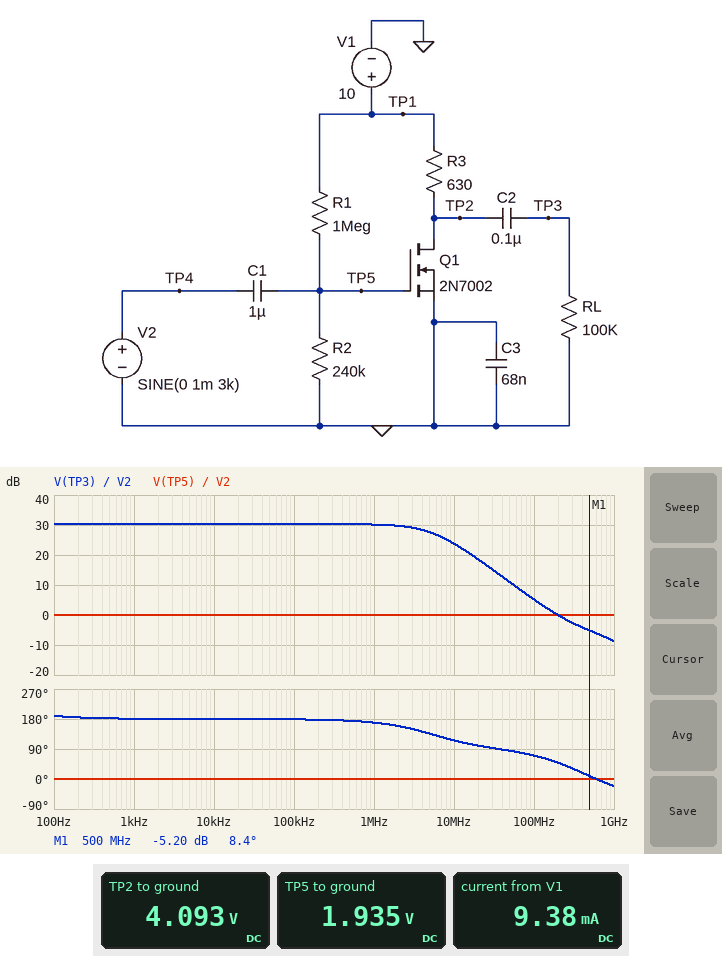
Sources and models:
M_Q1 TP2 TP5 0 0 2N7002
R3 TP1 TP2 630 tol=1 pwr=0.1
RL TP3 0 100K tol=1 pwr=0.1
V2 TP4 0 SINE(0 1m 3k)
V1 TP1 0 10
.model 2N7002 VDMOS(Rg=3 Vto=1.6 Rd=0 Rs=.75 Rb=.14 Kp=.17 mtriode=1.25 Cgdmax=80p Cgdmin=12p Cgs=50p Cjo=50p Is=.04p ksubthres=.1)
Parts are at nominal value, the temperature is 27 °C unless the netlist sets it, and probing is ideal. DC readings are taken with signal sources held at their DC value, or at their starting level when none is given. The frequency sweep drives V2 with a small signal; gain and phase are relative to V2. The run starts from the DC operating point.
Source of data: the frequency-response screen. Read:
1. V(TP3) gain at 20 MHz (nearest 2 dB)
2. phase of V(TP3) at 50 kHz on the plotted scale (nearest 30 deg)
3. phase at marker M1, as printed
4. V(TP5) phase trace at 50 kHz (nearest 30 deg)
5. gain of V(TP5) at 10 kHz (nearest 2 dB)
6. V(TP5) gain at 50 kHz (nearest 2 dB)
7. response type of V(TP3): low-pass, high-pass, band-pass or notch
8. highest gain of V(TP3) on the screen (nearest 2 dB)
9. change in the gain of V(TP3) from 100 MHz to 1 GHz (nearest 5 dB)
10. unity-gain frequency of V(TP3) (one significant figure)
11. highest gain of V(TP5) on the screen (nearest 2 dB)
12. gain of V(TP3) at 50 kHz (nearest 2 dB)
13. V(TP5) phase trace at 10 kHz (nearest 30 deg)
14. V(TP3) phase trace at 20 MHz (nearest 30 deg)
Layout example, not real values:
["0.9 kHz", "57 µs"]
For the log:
["18 dB", "180 deg", "8.4 deg", "0 deg", "0 dB", "0 dB", "low-pass", "30 dB", "-15 dB", "200 MHz", "0 dB", "30 dB", "0 deg", "90 deg"]
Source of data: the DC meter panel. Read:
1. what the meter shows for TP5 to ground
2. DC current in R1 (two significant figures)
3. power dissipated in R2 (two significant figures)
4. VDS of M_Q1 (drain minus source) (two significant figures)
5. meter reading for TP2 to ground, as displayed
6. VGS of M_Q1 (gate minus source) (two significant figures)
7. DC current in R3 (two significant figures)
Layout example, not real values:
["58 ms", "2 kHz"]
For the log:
["1.935 V", "8.1 µA", "16 µW", "4.1 V", "4.093 V", "1.9 V", "9.4 mA"]
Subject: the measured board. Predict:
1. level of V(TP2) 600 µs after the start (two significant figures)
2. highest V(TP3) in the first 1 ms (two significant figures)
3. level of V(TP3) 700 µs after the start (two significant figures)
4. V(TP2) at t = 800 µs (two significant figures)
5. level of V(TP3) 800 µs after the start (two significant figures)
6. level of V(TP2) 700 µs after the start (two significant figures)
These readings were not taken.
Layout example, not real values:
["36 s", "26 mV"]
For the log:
["4.1 V", "33 mV", "-19 mV", "4.1 V", "-19 mV", "4.1 V"]
